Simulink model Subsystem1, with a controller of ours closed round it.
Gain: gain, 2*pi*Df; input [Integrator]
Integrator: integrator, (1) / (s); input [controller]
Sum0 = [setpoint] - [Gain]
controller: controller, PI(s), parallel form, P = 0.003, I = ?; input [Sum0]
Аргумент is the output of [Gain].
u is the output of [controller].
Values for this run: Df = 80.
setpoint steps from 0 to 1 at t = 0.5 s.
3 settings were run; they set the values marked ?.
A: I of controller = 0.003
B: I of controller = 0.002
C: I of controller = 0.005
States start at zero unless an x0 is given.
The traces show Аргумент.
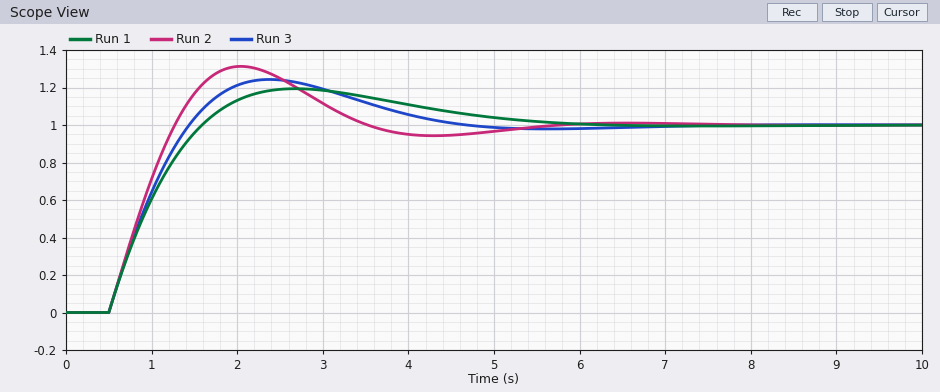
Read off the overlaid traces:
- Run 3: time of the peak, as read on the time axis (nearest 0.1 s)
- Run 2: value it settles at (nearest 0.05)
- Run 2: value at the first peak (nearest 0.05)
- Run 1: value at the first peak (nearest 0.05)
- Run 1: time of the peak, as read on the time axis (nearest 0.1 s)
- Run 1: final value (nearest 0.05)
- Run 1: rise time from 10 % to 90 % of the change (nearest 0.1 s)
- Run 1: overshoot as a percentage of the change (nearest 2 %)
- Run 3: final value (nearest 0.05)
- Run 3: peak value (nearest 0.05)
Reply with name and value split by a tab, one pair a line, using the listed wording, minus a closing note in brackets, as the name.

Run 3: time of the peak, as read on the time axis	2.4 s
Run 2: value it settles at	1.00
Run 2: value at the first peak	1.30
Run 1: value at the first peak	1.20
Run 1: time of the peak, as read on the time axis	2.7 s
Run 1: final value	1.00
Run 1: rise time from 10 % to 90 % of the change	0.8 s
Run 1: overshoot as a percentage of the change	20 %
Run 3: final value	1.00
Run 3: peak value	1.25
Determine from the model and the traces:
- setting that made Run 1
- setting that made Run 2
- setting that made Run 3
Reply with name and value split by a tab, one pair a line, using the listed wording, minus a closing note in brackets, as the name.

setting that made Run 1	B
setting that made Run 2	C
setting that made Run 3	A
